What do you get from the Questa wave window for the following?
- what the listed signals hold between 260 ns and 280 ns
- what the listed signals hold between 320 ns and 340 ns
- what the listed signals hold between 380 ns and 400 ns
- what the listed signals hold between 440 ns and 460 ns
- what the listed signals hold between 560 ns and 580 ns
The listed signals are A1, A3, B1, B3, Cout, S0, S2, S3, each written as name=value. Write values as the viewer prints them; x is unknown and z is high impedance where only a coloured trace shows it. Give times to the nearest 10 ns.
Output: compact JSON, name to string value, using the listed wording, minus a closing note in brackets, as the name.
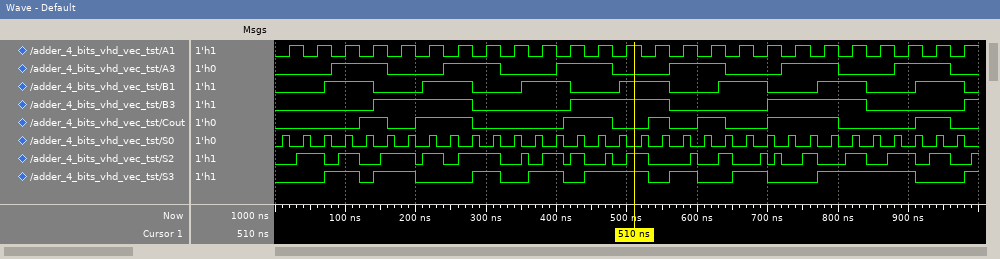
{"what the listed signals hold between 260 ns and 280 ns": "A1=1, A3=1, B1=1, B3=1, Cout=1, S0=0, S2=1, S3=0", "what the listed signals hold between 320 ns and 340 ns": "A1=0, A3=0, B1=0, B3=0, Cout=0, S0=0, S2=0, S3=0", "what the listed signals hold between 380 ns and 400 ns": "A1=1, A3=0, B1=1, B3=0, Cout=0, S0=0, S2=1, S3=1", "what the listed signals hold between 440 ns and 460 ns": "A1=0, A3=1, B1=0, B3=1, Cout=1, S0=0, S2=0, S3=1", "what the listed signals hold between 560 ns and 580 ns": "A1=0, A3=1, B1=0, B3=0, Cout=0, S0=0, S2=0, S3=1"}
